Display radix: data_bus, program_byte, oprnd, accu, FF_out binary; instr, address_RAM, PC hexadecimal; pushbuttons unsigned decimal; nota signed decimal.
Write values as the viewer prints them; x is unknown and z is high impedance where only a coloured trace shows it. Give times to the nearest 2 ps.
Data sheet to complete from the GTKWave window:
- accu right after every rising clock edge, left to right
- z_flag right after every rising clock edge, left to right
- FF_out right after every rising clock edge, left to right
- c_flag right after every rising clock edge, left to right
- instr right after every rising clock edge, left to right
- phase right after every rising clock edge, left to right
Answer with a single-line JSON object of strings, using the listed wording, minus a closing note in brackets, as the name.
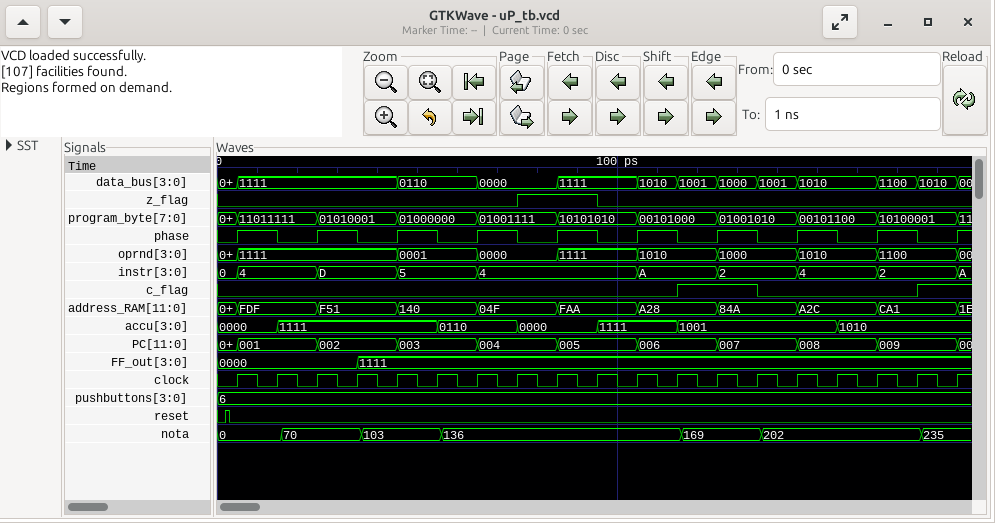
{"accu right after every rising clock edge, left to right": "0000, 1111, 1111, 1111, 1111, 0110, 0110, 0000, 0000, 1111, 1111, 1001, 1001, 1001, 1001, 1010, 1010, 1010, 1010", "z_flag right after every rising clock edge, left to right": "0 0 0 0 0 0 0 1 1 0 0 0 0 0 0 0 0 0 0", "FF_out right after every rising clock edge, left to right": "0000, 0000, 0000, 1111, 1111, 1111, 1111, 1111, 1111, 1111, 1111, 1111, 1111, 1111, 1111, 1111, 1111, 1111, 1111", "c_flag right after every rising clock edge, left to right": "0 0 0 0 0 0 0 0 0 0 0 1 1 0 0 0 0 1 1", "instr right after every rising clock edge, left to right": "4, 4, D, D, 5, 5, 4, 4, 4, 4, A, A, 2, 2, 4, 4, 2, 2, A", "phase right after every rising clock edge, left to right": "1 0 1 0 1 0 1 0 1 0 1 0 1 0 1 0 1 0 1"}
